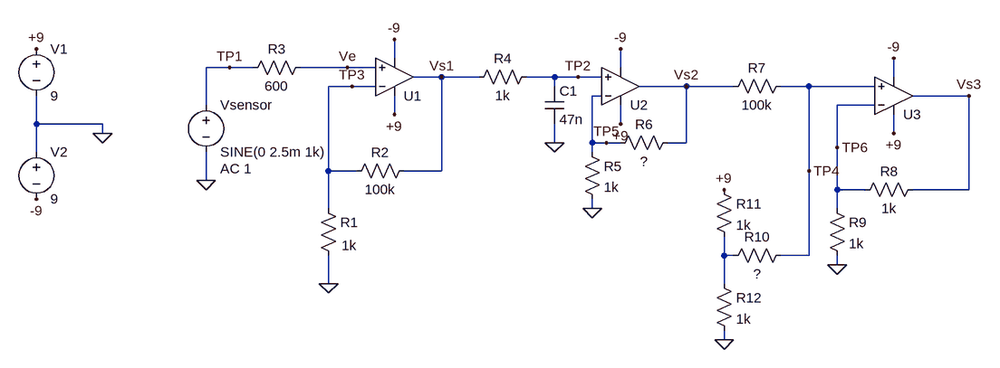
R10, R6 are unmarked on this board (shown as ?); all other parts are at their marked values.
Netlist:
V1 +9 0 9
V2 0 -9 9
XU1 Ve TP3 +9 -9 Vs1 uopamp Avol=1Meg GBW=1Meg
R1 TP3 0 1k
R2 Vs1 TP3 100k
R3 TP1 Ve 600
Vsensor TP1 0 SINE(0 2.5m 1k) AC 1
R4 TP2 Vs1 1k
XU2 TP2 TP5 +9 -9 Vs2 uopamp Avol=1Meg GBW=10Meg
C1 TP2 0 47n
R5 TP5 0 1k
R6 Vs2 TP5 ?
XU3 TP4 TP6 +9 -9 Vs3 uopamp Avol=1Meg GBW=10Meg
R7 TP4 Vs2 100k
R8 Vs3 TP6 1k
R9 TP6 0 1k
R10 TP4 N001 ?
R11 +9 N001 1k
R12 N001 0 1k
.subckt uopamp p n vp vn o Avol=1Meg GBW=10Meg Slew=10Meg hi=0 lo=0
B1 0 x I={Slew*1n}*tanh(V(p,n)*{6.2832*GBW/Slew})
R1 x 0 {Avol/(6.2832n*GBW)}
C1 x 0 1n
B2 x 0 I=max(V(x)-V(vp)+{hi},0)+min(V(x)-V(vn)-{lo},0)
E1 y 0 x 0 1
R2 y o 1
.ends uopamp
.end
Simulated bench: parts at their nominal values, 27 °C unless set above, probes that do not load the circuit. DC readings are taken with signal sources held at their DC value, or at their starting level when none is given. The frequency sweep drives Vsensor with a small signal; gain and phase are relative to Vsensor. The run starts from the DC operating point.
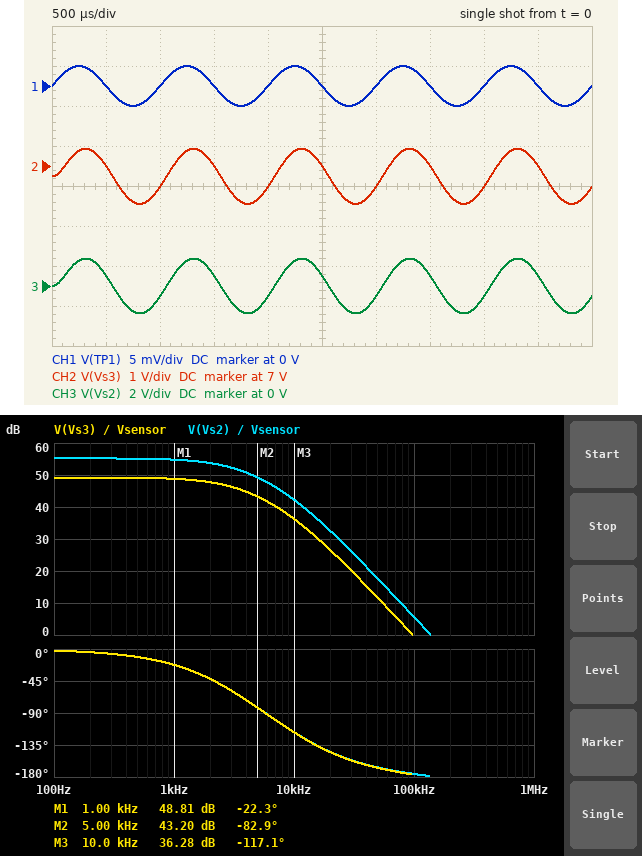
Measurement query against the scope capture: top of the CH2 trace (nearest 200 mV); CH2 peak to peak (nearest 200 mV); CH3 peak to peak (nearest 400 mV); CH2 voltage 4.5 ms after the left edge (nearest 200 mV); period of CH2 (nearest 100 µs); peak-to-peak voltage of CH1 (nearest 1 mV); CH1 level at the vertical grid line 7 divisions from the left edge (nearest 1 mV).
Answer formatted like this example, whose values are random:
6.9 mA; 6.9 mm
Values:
7.4 V; 1.4 V; 2.8 V; 7.0 V; 1.0 ms; 5 mV; 0 V
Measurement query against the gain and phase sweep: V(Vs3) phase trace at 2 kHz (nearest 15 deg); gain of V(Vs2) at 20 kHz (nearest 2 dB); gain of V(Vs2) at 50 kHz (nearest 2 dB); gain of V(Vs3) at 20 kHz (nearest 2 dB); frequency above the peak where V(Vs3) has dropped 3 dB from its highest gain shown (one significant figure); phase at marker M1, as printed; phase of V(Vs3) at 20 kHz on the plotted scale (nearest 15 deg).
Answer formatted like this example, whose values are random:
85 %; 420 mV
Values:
-45 deg; 32 dB; 18 dB; 26 dB; 3 kHz; -22.3 deg; -150 deg
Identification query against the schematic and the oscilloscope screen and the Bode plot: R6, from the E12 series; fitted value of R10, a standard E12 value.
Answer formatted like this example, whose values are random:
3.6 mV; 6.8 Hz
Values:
4.7 kΩ; 33 kΩ
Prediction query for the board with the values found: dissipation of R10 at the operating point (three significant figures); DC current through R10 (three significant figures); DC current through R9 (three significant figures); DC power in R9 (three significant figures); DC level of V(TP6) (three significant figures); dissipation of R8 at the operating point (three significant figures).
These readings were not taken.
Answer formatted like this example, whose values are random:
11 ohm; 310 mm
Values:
37.5 µW; 33.7 µA; 3.37 mA; 11.4 mW; 3.37 V; 11.4 mW
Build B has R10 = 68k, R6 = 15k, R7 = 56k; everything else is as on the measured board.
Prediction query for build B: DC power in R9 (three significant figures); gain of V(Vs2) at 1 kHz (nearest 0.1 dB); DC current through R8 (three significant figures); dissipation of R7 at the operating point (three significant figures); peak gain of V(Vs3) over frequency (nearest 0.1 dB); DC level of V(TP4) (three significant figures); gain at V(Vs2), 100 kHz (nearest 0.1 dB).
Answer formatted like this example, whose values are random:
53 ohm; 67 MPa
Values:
4.10 mW; 63.8 dB; 2.02 mA; 73.2 µW; 65.0 dB; 2.02 V; 14.5 dB
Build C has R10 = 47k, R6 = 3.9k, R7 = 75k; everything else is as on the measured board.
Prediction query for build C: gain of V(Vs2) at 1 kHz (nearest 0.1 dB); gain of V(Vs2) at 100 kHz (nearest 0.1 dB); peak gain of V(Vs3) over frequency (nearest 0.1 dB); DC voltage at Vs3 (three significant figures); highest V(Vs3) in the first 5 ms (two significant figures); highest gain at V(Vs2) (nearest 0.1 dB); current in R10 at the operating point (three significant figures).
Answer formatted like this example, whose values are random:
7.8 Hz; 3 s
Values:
53.5 dB; 4.3 dB; 51.7 dB; 5.51 V; 6.4 V; 53.9 dB; 36.7 µA
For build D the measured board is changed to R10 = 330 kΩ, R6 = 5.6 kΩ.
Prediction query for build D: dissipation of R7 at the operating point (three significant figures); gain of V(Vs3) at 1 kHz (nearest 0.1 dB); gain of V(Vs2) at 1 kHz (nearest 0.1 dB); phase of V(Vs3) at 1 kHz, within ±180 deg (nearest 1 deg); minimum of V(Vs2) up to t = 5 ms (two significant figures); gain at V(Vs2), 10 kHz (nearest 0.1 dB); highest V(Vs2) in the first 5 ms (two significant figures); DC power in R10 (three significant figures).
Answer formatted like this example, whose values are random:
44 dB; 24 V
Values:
10.9 µW; 59.8 dB; 56.1 dB; -22 deg; -1.6 V; 43.5 dB; 1.6 V; 36.1 µW
